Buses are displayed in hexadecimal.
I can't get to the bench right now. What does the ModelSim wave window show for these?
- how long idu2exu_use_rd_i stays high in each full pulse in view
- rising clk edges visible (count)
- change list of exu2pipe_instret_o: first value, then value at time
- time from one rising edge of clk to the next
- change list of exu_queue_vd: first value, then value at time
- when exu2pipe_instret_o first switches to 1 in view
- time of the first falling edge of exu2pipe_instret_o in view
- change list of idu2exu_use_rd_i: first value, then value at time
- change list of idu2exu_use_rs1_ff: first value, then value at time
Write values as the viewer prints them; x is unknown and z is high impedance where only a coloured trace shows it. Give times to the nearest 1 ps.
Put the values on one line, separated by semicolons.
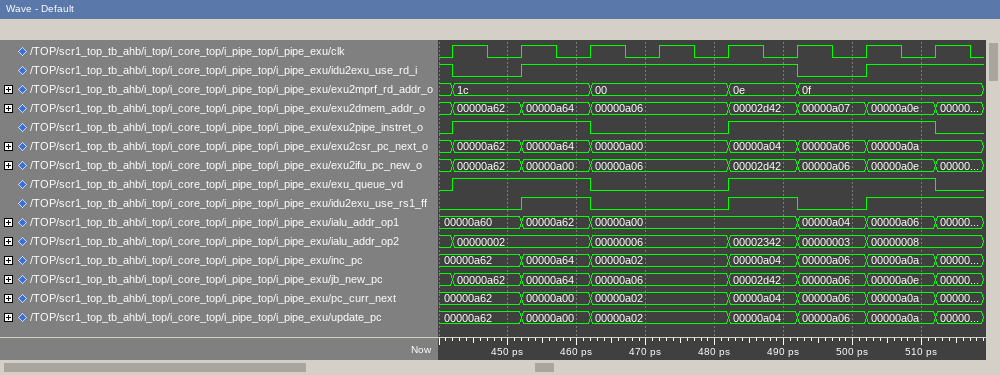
40 ps; 8; 0, 1 at 442 ps, 0 at 462 ps, 1 at 482 ps, 0 at 512 ps; 10 ps; 0, 1 at 442 ps, 0 at 462 ps, 1 at 482 ps, 0 at 512 ps; 442 ps; 462 ps; 1, 0 at 442 ps, 1 at 452 ps, 0 at 492 ps, 1 at 502 ps; 0, 1 at 452 ps, 0 at 462 ps, 1 at 482 ps, 0 at 492 ps, 1 at 502 ps
